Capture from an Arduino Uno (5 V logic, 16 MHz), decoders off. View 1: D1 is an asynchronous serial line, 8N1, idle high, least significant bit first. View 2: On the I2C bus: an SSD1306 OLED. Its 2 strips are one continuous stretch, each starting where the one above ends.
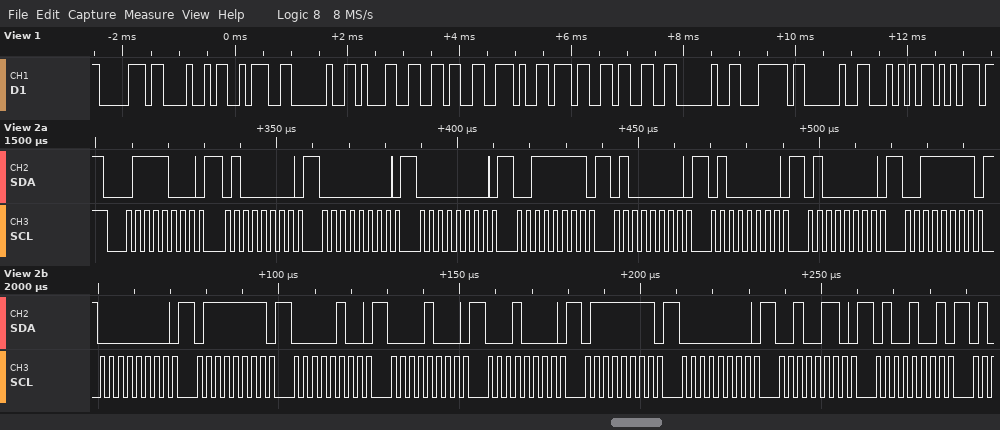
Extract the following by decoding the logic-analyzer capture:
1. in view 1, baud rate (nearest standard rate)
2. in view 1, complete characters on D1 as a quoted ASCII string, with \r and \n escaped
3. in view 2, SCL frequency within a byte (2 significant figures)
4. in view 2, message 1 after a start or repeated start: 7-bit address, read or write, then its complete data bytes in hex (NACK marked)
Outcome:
9600 baud
"pH: 16.73 | Tu"
400 kHz
0x3C write: 40 00 00 3F 40 40 40 3F 00 7F 04 08 10 7F 00 26 49
